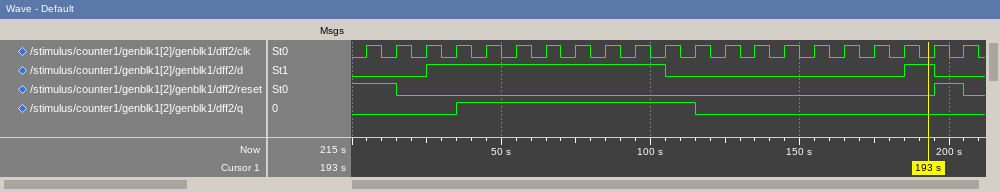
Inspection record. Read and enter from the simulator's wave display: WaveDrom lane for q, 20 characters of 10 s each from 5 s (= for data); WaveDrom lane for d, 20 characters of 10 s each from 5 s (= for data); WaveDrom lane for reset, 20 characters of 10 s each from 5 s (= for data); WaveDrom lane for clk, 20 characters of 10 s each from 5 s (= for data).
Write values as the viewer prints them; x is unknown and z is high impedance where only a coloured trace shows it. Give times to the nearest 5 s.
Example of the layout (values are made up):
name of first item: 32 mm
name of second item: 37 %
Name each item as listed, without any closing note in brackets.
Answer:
WaveDrom lane for q, 20 characters of 10 s each from 5 s: {name: 'q', wave: '0..1.......0........'}
WaveDrom lane for d, 20 characters of 10 s each from 5 s: {name: 'd', wave: '0.1.......0.......10'}
WaveDrom lane for reset, 20 characters of 10 s each from 5 s: {name: 'reset', wave: '10.................1'}
WaveDrom lane for clk, 20 characters of 10 s each from 5 s: {name: 'clk', wave: 'p...................'}
